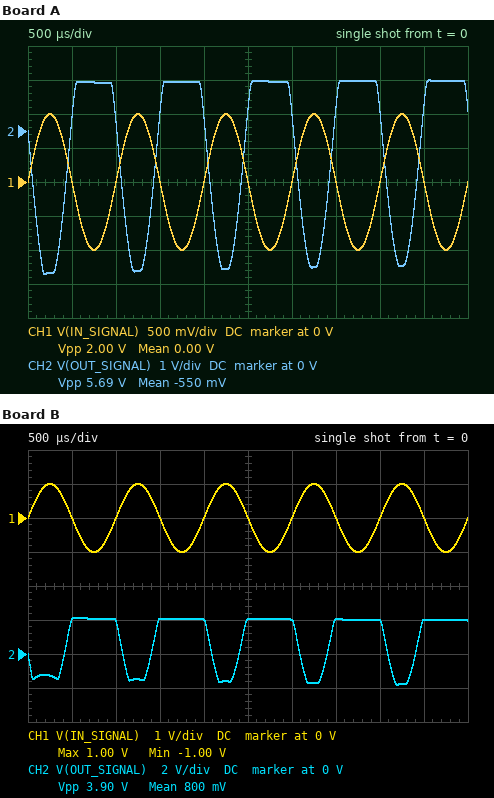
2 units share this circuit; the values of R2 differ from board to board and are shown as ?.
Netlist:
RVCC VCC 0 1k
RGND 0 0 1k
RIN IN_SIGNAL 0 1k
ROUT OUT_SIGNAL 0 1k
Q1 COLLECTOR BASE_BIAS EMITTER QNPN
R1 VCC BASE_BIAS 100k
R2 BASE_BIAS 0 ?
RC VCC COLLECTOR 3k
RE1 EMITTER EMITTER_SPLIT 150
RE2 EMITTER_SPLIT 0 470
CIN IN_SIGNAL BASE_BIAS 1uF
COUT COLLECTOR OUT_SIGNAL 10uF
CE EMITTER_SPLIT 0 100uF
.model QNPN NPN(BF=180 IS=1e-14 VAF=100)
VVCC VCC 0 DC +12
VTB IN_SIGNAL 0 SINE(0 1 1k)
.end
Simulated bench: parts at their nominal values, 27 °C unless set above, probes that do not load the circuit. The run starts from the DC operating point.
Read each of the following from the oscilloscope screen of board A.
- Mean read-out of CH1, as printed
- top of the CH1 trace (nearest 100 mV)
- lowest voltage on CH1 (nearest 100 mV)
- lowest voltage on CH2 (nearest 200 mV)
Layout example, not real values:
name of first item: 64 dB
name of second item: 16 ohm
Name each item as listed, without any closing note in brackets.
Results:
Mean read-out of CH1, as printed: 0.00 V
top of the CH1 trace: 1.0 V
lowest voltage on CH1: -1.0 V
lowest voltage on CH2: -4.2 V
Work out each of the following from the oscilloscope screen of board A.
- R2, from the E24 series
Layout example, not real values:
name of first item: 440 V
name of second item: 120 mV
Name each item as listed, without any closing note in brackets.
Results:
R2, from the E24 series: 20 kΩ
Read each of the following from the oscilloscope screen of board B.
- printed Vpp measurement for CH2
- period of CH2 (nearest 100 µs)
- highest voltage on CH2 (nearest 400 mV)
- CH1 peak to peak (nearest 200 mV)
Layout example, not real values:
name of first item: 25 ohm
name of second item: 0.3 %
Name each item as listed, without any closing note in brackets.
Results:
printed Vpp measurement for CH2: 3.90 V
period of CH2: 1.0 ms
highest voltage on CH2: 2.0 V
CH1 peak to peak: 2.0 V
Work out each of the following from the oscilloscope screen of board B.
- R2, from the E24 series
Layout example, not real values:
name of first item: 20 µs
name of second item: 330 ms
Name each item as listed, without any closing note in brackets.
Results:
R2, from the E24 series: 30 kΩ
